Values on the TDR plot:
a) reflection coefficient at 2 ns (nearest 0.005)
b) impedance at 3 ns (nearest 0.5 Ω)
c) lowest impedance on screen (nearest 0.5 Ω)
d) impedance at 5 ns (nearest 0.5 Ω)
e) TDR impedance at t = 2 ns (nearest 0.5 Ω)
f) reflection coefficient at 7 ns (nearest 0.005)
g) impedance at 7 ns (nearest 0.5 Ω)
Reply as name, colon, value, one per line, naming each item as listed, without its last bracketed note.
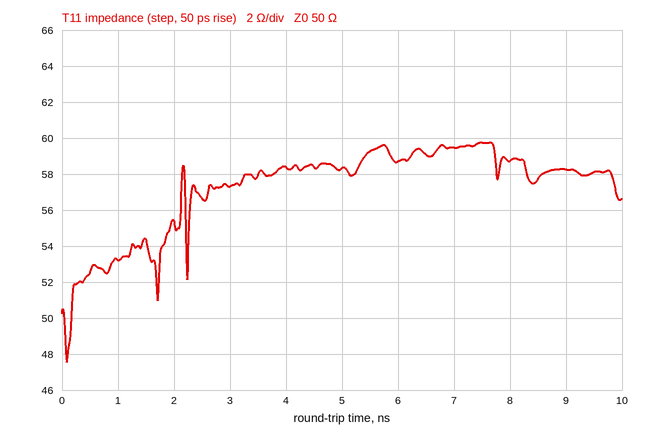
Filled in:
reflection coefficient at 2 ns: +0.050
impedance at 3 ns: 57.5 Ω
lowest impedance on screen: 47.5 Ω
impedance at 5 ns: 58.5 Ω
TDR impedance at t = 2 ns: 55.5 Ω
reflection coefficient at 7 ns: +0.085
impedance at 7 ns: 59.5 Ω
